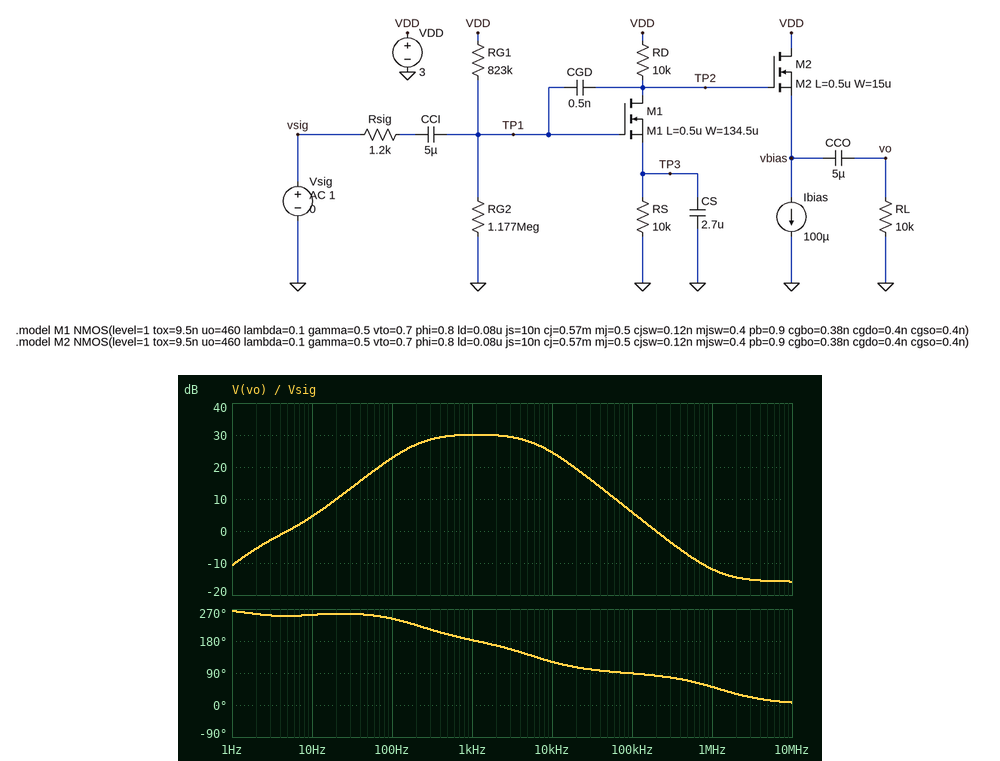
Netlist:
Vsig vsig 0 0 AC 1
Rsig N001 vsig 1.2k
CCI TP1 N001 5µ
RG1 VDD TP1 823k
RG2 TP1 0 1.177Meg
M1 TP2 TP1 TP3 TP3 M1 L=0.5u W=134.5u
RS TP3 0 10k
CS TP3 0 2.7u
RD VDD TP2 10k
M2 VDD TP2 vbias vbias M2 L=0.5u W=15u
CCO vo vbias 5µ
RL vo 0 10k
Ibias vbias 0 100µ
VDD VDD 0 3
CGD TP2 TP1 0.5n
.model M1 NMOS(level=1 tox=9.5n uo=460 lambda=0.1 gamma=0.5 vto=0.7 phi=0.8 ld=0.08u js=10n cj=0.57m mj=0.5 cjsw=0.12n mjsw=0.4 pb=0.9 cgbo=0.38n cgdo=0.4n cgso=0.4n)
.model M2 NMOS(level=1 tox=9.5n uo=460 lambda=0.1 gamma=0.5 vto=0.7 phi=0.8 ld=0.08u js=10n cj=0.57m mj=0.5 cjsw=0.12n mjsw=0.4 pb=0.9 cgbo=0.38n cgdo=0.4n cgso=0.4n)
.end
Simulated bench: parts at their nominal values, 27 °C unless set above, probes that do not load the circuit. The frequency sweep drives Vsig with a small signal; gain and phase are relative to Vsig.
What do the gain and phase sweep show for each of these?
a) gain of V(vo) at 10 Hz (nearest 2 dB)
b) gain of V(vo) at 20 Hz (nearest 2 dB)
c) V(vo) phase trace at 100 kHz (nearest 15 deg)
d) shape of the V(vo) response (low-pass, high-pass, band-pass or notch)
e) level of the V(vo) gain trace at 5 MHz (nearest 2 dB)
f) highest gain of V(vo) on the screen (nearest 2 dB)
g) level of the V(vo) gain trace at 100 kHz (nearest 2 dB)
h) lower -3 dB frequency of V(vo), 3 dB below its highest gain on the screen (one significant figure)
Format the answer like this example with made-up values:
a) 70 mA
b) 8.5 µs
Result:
a) 4 dB
b) 10 dB
c) 90 deg
d) band-pass
e) -16 dB
f) 30 dB
g) 6 dB
h) 200 Hz
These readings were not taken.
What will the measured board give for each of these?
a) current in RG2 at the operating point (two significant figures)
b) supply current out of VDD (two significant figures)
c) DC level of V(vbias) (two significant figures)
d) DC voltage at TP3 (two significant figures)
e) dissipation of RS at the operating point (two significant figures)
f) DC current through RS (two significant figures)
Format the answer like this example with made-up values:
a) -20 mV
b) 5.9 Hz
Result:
a) 1.5 µA
b) 200 µA
c) 1.1 V
d) 1.0 V
e) 100 µW
f) 100 µA
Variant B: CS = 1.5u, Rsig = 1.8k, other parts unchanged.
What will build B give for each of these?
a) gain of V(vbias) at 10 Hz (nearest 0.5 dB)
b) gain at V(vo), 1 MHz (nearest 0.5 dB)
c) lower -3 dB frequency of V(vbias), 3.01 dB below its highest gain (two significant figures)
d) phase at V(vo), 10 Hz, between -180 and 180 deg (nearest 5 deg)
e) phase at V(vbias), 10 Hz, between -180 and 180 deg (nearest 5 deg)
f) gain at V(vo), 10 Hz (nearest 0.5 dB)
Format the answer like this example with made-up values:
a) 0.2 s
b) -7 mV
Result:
a) 2.0 dB
b) -15.0 dB
c) 350 Hz
d) -120 deg
e) -140 deg
f) 1.5 dB
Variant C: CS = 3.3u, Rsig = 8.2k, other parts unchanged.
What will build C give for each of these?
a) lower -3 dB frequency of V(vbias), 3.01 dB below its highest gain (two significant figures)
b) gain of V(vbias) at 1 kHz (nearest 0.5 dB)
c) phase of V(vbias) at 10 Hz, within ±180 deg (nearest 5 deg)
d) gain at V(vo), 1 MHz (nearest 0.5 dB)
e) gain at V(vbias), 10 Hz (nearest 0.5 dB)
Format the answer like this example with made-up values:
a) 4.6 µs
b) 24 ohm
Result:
a) 150 Hz
b) 28.0 dB
c) -120 deg
d) -27.0 dB
e) 6.0 dB
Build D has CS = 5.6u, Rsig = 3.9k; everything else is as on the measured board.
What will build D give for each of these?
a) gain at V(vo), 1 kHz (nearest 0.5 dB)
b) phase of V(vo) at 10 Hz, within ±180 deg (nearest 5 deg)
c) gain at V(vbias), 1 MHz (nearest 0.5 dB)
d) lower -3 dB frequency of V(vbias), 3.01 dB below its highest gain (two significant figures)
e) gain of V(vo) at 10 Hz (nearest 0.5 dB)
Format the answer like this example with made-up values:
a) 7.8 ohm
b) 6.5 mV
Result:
a) 29.5 dB
b) -95 deg
c) -21.0 dB
d) 97 Hz
e) 10.0 dB
